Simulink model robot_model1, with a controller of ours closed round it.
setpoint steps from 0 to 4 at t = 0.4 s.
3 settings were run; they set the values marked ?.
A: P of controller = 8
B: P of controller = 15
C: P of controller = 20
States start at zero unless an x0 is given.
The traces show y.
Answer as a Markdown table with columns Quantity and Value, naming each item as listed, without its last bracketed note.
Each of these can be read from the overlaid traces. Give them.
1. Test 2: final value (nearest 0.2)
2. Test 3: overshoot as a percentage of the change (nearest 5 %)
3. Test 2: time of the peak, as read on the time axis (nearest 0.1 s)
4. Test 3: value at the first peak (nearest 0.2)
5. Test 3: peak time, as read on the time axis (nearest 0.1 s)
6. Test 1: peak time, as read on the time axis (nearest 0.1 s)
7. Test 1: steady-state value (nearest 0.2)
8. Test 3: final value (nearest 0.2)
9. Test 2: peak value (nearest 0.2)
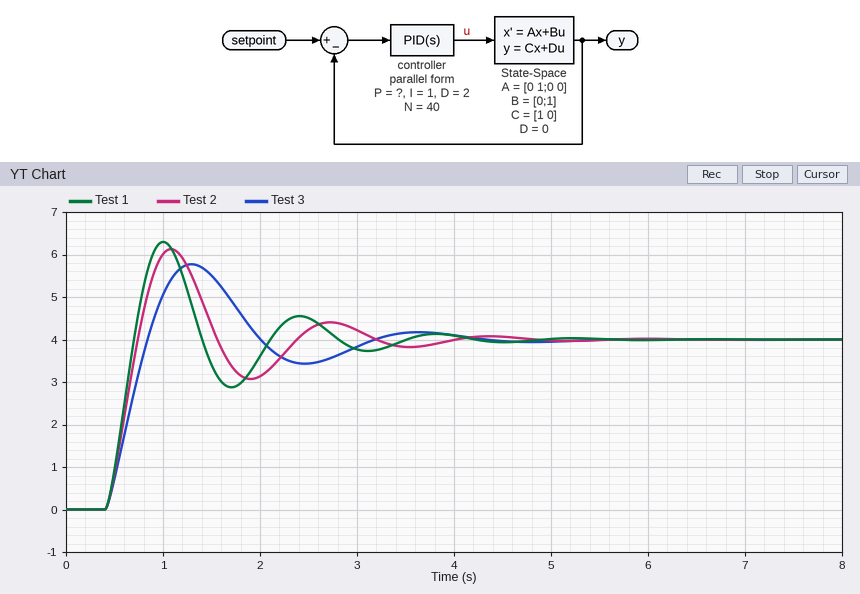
| Quantity | Value |
|---|---|
| Test 2: final value | 4.0 |
| Test 3: overshoot as a percentage of the change | 45 % |
| Test 2: time of the peak, as read on the time axis | 1.1 s |
| Test 3: value at the first peak | 5.8 |
| Test 3: peak time, as read on the time axis | 1.3 s |
| Test 1: peak time, as read on the time axis | 1.0 s |
| Test 1: steady-state value | 4.0 |
| Test 3: final value | 4.0 |
| Test 2: peak value | 6.2 |
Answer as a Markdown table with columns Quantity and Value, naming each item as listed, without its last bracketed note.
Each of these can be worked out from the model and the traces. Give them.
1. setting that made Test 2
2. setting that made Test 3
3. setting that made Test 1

| Quantity | Value |
|---|---|
| setting that made Test 2 | B |
| setting that made Test 3 | A |
| setting that made Test 1 | C |
